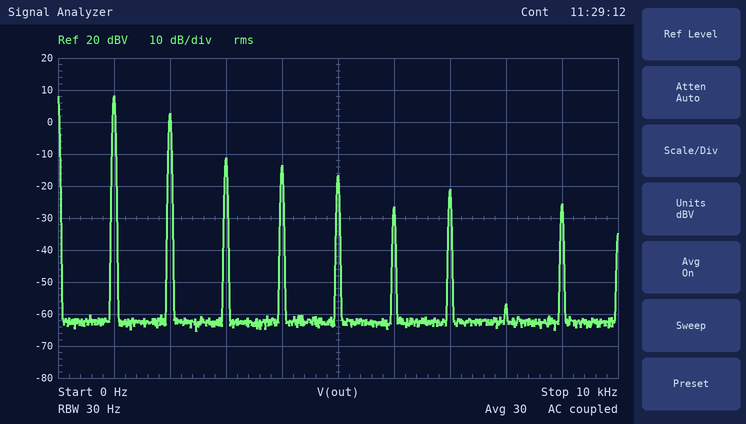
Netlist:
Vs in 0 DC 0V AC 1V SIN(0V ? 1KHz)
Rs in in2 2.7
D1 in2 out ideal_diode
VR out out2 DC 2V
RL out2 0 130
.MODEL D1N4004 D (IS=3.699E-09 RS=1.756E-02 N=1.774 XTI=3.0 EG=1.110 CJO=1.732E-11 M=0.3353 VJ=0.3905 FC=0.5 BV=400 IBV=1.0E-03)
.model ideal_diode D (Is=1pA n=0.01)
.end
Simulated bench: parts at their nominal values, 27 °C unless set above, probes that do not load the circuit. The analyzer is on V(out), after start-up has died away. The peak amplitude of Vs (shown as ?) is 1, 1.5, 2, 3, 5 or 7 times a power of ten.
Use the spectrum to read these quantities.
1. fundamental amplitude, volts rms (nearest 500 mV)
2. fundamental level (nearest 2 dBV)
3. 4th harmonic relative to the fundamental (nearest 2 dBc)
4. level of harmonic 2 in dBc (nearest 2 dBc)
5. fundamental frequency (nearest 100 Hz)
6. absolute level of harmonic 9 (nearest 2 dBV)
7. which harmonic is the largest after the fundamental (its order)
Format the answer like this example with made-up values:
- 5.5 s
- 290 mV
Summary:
- 2.5 V
- 8 dBV
- -22 dBc
- -6 dBc
- 1.0 kHz
- -26 dBV
- 2
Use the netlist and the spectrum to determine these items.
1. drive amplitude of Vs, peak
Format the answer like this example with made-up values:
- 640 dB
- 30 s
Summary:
- 10 V
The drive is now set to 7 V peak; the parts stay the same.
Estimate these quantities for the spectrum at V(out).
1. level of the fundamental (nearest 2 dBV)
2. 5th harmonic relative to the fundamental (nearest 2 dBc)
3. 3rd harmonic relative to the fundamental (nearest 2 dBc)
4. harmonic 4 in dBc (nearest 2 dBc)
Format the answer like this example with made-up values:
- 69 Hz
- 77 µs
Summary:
- 4 dBV
- -22 dBc
- -16 dBc
- -24 dBc
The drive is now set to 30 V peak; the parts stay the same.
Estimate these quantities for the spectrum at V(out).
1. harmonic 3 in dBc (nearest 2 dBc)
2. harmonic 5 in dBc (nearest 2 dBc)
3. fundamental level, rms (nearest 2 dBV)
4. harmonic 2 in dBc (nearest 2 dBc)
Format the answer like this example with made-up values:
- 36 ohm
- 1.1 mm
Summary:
- -30 dBc
- -34 dBc
- 20 dBV
- -6 dBc
